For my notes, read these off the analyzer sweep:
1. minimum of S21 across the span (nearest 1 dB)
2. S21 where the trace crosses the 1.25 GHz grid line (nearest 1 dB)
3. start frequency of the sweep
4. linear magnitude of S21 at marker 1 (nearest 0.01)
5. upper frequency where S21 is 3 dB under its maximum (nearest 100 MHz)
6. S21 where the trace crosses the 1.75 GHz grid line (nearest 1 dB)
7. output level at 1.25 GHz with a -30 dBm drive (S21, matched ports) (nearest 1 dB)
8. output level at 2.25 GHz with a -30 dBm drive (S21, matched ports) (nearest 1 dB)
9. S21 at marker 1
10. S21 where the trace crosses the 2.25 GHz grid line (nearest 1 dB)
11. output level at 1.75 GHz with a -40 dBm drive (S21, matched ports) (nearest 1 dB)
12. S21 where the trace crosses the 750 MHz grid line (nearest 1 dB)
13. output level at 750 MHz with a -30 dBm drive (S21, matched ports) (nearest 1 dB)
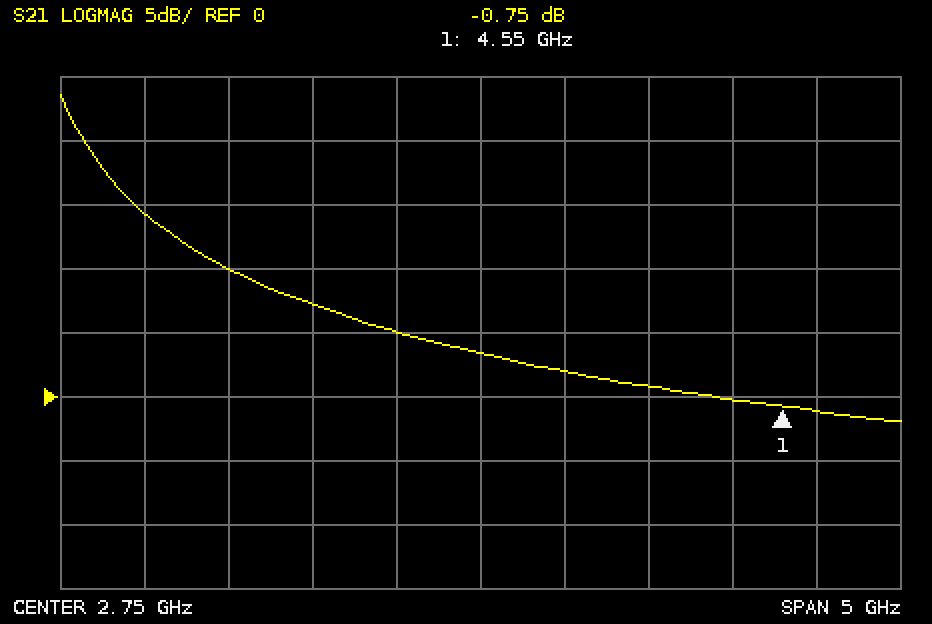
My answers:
-2 dB
10 dB
250 MHz
0.92
400 MHz
7 dB
-20 dBm
-25 dBm
-0.75 dB
5 dB
-33 dBm
14 dB
-16 dBm
